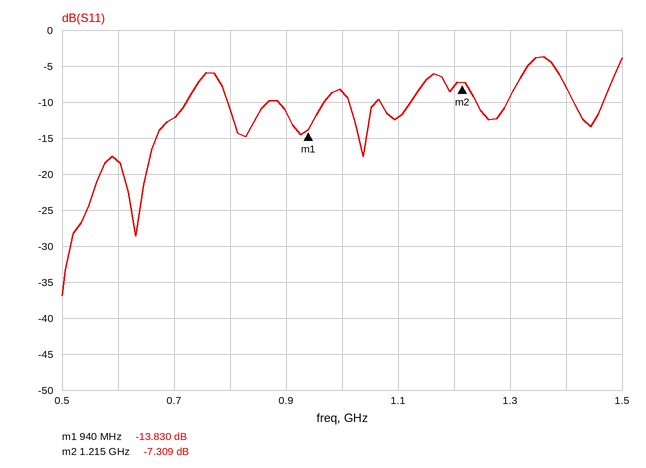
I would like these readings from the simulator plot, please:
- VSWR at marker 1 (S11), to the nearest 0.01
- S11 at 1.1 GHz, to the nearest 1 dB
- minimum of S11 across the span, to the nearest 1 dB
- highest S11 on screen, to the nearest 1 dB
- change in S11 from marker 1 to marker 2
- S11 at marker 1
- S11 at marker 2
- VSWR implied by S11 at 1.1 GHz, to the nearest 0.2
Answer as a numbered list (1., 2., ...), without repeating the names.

1. 1.51
2. -12 dB
3. -37 dB
4. -4 dB
5. 6.521 dB
6. -13.830 dB
7. -7.309 dB
8. 1.6
